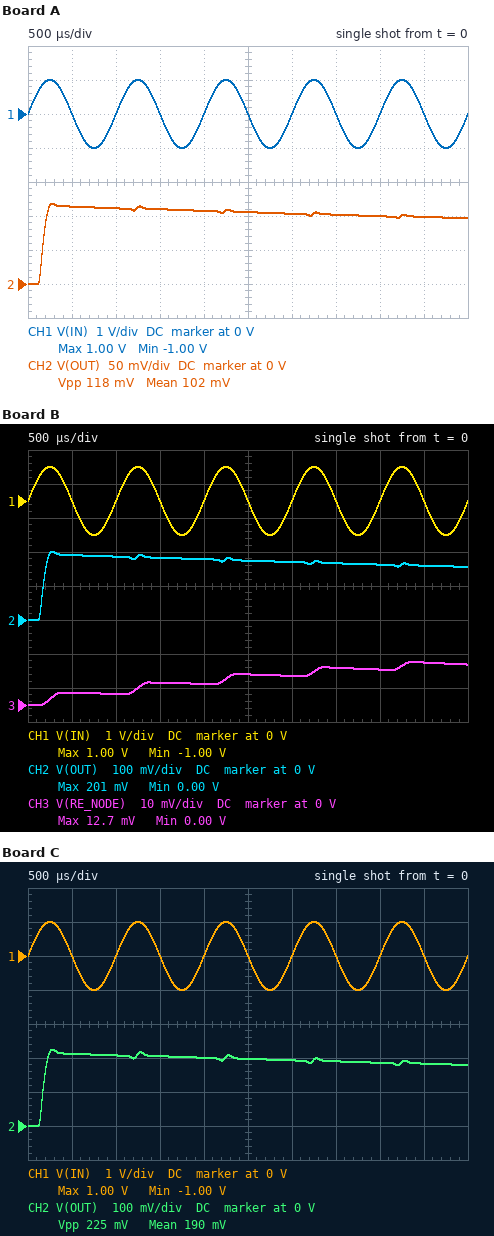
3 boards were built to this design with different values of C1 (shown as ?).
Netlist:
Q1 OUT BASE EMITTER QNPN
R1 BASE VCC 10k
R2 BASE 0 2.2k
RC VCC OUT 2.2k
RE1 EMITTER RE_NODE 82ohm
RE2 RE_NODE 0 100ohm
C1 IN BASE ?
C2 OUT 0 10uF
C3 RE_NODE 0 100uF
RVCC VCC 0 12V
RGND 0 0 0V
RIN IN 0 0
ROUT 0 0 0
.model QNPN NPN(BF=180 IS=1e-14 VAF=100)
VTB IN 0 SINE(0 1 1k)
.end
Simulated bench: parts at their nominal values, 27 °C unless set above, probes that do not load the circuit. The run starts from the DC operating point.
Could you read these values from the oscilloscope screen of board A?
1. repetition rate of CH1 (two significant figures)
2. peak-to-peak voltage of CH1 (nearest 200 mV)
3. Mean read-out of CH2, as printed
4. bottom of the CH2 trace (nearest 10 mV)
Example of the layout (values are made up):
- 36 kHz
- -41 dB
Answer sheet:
- 1.0 kHz
- 2.0 V
- 102 mV
- 0 V
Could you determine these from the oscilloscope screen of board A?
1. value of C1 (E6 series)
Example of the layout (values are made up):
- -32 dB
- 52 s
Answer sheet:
- 6.8 µF
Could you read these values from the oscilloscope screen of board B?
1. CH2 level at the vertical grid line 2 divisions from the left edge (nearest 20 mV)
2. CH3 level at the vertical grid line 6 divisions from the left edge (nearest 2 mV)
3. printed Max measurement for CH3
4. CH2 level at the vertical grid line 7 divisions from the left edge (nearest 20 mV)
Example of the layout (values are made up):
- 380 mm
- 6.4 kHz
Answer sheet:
- 180 mV
- 8 mV
- 12.7 mV
- 160 mV
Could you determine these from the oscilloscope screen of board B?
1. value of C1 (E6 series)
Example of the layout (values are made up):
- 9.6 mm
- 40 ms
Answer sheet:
- 22 µF
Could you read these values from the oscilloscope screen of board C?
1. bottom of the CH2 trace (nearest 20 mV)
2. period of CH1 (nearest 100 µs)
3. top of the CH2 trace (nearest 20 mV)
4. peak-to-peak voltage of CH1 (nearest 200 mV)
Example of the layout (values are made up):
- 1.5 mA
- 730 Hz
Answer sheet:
- 0 V
- 1.0 ms
- 220 mV
- 2.0 V
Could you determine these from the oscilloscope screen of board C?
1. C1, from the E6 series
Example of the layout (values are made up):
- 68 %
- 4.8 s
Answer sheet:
- 33 µF
